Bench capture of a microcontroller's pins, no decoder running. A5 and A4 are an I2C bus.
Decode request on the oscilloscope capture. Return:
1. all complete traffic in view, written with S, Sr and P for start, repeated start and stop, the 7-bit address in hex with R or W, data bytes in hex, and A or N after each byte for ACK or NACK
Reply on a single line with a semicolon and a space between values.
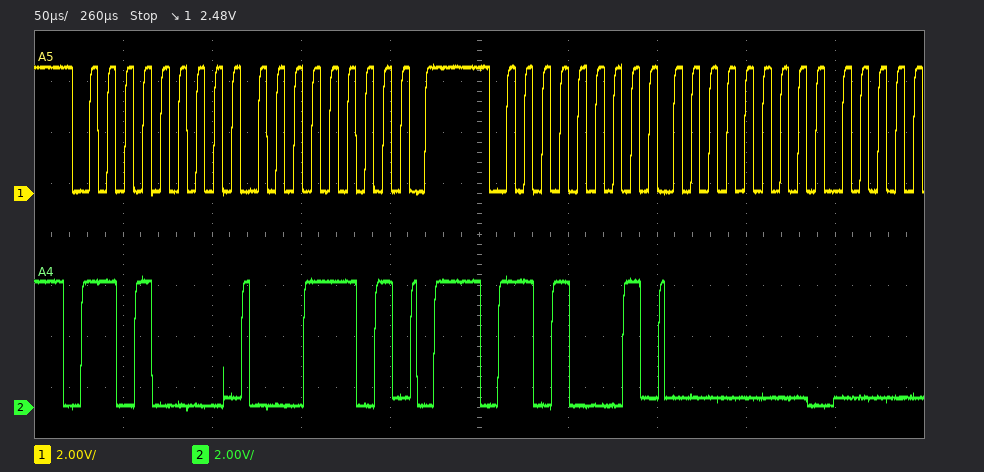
S 68W A 1D A P S 68R A 00 A
